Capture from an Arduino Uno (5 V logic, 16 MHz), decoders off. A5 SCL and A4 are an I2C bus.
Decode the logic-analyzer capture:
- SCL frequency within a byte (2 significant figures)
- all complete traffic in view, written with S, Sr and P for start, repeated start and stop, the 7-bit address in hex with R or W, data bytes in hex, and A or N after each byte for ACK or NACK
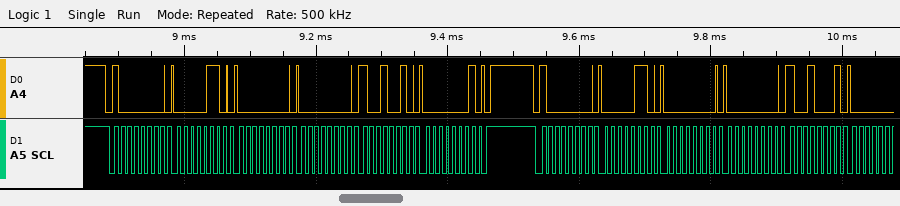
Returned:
100 kHz
S 40W A 06 A 00 A 00 A 92 A 01 A P S 40W A 06 A 00 A 00 A 91 A
